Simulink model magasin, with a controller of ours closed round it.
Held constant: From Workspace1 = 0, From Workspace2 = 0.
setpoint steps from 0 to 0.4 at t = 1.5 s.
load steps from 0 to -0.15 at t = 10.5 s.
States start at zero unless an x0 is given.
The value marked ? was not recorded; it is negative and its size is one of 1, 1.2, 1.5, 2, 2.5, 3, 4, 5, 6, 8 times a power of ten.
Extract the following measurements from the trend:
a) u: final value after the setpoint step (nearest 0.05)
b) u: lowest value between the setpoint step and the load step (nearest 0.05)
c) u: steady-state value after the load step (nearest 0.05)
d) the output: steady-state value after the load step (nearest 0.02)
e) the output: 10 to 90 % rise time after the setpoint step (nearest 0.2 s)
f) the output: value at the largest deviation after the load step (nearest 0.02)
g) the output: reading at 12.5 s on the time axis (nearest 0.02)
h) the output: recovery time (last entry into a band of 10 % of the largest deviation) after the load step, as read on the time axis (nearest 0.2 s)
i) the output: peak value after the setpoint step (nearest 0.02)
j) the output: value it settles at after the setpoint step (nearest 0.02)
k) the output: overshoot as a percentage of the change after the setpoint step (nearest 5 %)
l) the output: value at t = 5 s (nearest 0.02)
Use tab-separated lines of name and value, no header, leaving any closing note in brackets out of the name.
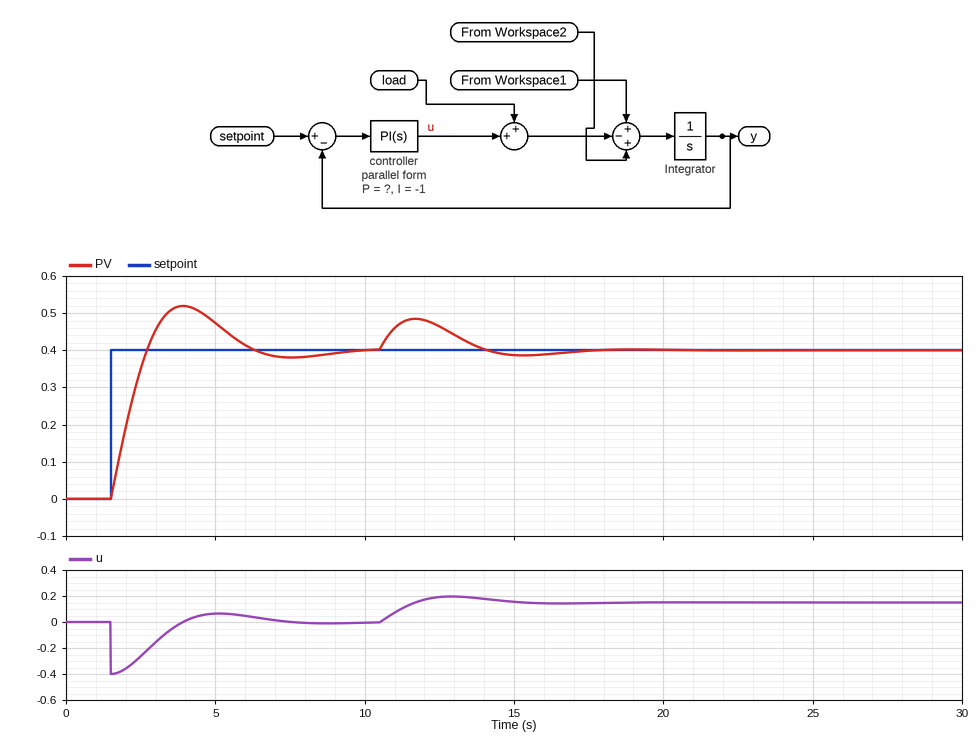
u: final value after the setpoint step	0.00
u: lowest value between the setpoint step and the load step	-0.40
u: steady-state value after the load step	0.15
the output: steady-state value after the load step	0.40
the output: 10 to 90 % rise time after the setpoint step	1.0 s
the output: value at the largest deviation after the load step	0.48
the output: reading at 12.5 s on the time axis	0.46
the output: recovery time (last entry into a band of 10 % of the largest deviation) after the load step, as read on the time axis	16.4 s
the output: peak value after the setpoint step	0.52
the output: value it settles at after the setpoint step	0.40
the output: overshoot as a percentage of the change after the setpoint step	30 %
the output: value at t = 5 s	0.48
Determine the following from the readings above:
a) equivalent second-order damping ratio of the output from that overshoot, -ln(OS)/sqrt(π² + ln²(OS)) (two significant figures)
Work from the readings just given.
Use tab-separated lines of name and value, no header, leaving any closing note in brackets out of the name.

equivalent second-order damping ratio of the output from that overshoot, -ln(OS)/sqrt(π² + ln²(OS))	0.36
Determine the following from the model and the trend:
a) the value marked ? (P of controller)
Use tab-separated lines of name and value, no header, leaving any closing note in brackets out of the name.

the value marked ?	-1
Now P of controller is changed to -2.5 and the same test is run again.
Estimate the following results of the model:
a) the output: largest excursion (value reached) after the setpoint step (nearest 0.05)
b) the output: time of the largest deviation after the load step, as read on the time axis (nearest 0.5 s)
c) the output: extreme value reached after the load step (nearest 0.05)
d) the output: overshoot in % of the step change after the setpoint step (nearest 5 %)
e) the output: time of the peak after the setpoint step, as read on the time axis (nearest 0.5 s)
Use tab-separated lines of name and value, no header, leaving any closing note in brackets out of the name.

the output: largest excursion (value reached) after the setpoint step	0.45
the output: time of the largest deviation after the load step, as read on the time axis	11.5 s
the output: extreme value reached after the load step	0.45
the output: overshoot in % of the step change after the setpoint step	10 %
the output: time of the peak after the setpoint step, as read on the time axis	3.5 s
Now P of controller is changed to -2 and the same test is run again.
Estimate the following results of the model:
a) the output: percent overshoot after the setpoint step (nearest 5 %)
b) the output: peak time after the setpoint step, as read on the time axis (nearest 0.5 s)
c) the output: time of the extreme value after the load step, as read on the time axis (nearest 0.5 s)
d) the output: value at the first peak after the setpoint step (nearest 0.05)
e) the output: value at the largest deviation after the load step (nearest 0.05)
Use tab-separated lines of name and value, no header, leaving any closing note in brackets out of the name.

the output: percent overshoot after the setpoint step	15 %
the output: peak time after the setpoint step, as read on the time axis	3.5 s
the output: time of the extreme value after the load step, as read on the time axis	11.5 s
the output: value at the first peak after the setpoint step	0.45
the output: value at the largest deviation after the load step	0.45
